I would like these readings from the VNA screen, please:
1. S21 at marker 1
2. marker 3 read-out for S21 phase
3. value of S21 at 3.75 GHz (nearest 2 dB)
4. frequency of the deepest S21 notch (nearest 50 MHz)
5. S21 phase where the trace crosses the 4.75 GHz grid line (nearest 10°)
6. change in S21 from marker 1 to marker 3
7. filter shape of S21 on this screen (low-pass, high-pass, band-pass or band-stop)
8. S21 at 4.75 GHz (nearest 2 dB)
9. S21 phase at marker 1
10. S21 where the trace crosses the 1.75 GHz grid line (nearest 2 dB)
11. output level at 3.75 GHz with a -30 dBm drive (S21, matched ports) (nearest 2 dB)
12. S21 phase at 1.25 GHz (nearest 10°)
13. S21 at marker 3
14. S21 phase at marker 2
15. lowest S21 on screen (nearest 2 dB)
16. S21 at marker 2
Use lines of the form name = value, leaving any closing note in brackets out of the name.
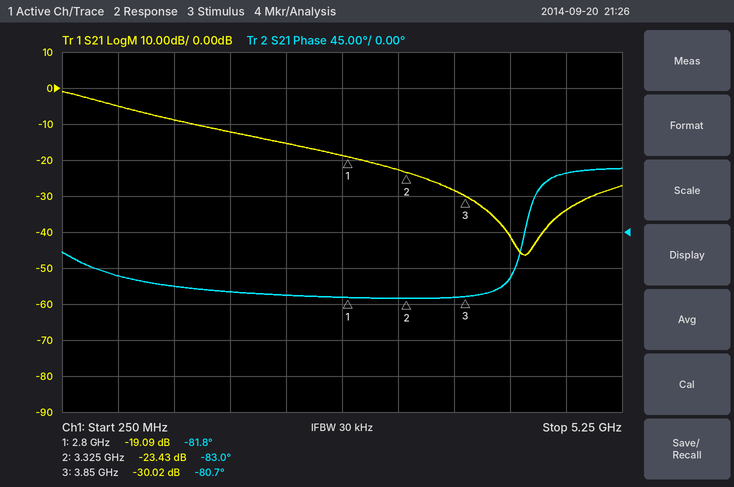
S21 at marker 1 = -19.09 dB
marker 3 read-out for S21 phase = -80.7°
value of S21 at 3.75 GHz = -28 dB
frequency of the deepest S21 notch = 4.40 GHz
S21 phase where the trace crosses the 4.75 GHz grid line = 70°
change in S21 from marker 1 to marker 3 = -10.93 dB
filter shape of S21 on this screen = low-pass
S21 at 4.75 GHz = -34 dB
S21 phase at marker 1 = -81.8°
S21 where the trace crosses the 1.75 GHz grid line = -12 dB
output level at 3.75 GHz with a -30 dBm drive (S21, matched ports) = -58 dBm
S21 phase at 1.25 GHz = -70°
S21 at marker 3 = -30.02 dB
S21 phase at marker 2 = -83.0°
lowest S21 on screen = -46 dB
S21 at marker 2 = -23.43 dB
